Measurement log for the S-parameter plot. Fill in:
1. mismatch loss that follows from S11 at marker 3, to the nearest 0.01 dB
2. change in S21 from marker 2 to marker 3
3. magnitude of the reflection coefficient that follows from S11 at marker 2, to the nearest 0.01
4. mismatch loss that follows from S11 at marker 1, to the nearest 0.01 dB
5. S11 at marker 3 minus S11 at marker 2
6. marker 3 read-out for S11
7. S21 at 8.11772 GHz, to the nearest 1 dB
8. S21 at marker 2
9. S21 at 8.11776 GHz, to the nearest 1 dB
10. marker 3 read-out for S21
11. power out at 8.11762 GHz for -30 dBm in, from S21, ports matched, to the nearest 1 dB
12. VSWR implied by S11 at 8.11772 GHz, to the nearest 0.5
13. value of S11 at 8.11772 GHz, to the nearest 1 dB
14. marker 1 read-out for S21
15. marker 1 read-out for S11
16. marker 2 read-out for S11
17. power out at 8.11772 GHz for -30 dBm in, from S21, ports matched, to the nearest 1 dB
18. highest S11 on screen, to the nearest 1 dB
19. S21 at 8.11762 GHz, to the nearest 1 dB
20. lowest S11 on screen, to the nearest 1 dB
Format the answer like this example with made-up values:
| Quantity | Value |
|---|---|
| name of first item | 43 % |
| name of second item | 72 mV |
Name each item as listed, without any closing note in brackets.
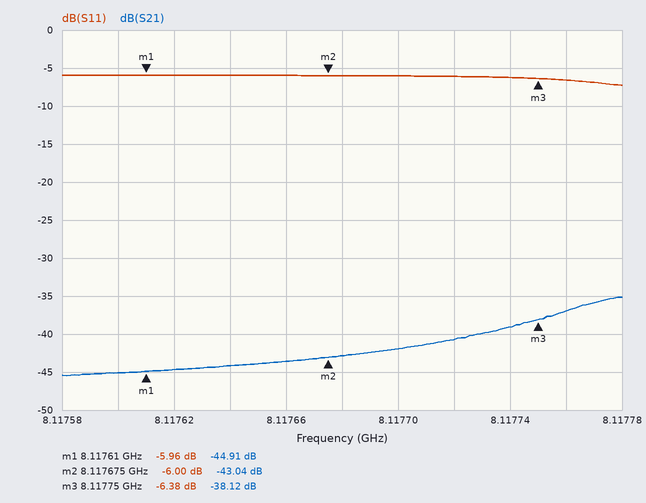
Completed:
| Quantity | Value |
|---|---|
| mismatch loss that follows from S11 at marker 3, to the nearest 0.01 dB | 1.14 dB |
| change in S21 from marker 2 to marker 3 | 4.92 dB |
| magnitude of the reflection coefficient that follows from S11 at marker 2, to the nearest 0.01 | 0.50 |
| mismatch loss that follows from S11 at marker 1, to the nearest 0.01 dB | 1.27 dB |
| S11 at marker 3 minus S11 at marker 2 | -0.38 dB |
| marker 3 read-out for S11 | -6.38 dB |
| S21 at 8.11772 GHz, to the nearest 1 dB | -41 dB |
| S21 at marker 2 | -43.04 dB |
| S21 at 8.11776 GHz, to the nearest 1 dB | -37 dB |
| marker 3 read-out for S21 | -38.12 dB |
| power out at 8.11762 GHz for -30 dBm in, from S21, ports matched, to the nearest 1 dB | -75 dBm |
| VSWR implied by S11 at 8.11772 GHz, to the nearest 0.5 | 3.0 |
| value of S11 at 8.11772 GHz, to the nearest 1 dB | -6 dB |
| marker 1 read-out for S21 | -44.91 dB |
| marker 1 read-out for S11 | -5.96 dB |
| marker 2 read-out for S11 | -6.00 dB |
| power out at 8.11772 GHz for -30 dBm in, from S21, ports matched, to the nearest 1 dB | -71 dBm |
| highest S11 on screen, to the nearest 1 dB | -6 dB |
| S21 at 8.11762 GHz, to the nearest 1 dB | -45 dB |
| lowest S11 on screen, to the nearest 1 dB | -7 dB |
